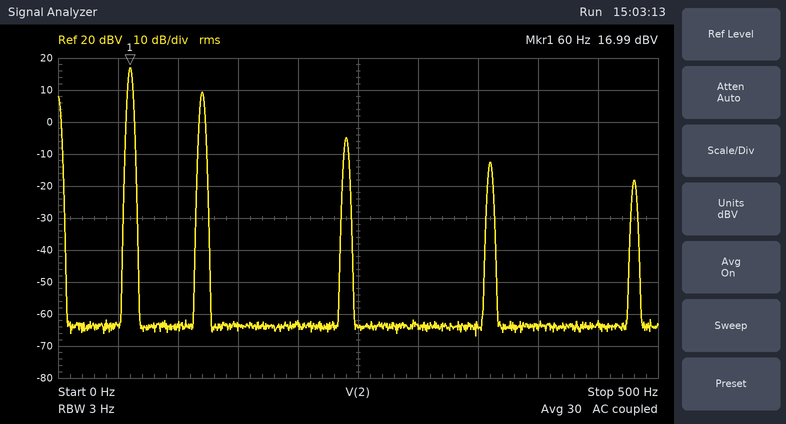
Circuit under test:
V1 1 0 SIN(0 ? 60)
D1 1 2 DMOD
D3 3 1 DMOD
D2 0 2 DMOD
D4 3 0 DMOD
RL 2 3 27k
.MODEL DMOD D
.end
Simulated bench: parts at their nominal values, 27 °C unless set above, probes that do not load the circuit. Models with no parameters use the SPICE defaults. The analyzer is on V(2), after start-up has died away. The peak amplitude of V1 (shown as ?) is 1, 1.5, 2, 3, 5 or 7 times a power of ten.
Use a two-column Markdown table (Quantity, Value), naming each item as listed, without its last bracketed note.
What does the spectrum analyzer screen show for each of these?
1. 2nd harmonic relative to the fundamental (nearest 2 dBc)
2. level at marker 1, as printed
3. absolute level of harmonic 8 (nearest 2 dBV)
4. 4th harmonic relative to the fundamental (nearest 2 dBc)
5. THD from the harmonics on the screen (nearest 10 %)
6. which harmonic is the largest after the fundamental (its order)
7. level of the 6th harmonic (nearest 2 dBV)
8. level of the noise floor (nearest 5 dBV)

| Quantity | Value |
|---|---|
| 2nd harmonic relative to the fundamental | -8 dBc |
| level at marker 1, as printed | 16.99 dBV |
| absolute level of harmonic 8 | -18 dBV |
| 4th harmonic relative to the fundamental | -22 dBc |
| THD from the harmonics on the screen | 40 % |
| which harmonic is the largest after the fundamental | 2 |
| level of the 6th harmonic | -12 dBV |
| level of the noise floor | -65 dBV |
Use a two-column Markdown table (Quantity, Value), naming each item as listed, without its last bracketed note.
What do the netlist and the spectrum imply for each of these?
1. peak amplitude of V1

| Quantity | Value |
|---|---|
| peak amplitude of V1 | 20 V |
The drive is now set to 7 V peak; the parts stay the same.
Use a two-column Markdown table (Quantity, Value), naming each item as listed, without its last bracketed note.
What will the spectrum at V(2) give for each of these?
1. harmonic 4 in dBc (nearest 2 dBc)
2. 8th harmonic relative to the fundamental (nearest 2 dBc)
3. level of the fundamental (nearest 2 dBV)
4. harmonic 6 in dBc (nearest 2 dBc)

| Quantity | Value |
|---|---|
| harmonic 4 in dBc | -24 dBc |
| 8th harmonic relative to the fundamental | -44 dBc |
| level of the fundamental | 8 dBV |
| harmonic 6 in dBc | -34 dBc |
